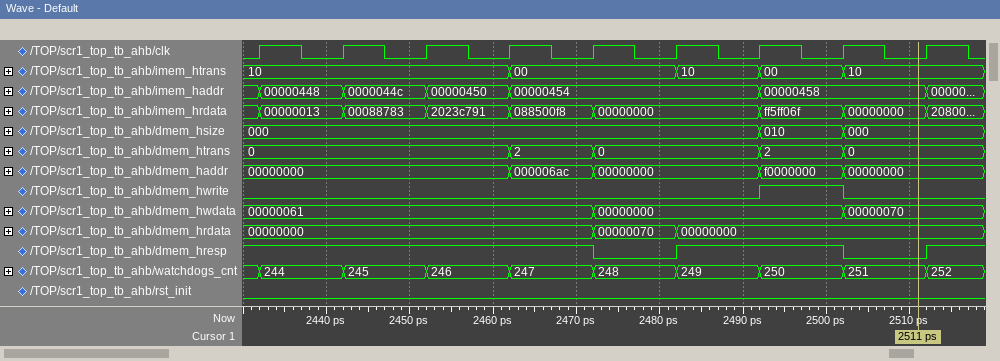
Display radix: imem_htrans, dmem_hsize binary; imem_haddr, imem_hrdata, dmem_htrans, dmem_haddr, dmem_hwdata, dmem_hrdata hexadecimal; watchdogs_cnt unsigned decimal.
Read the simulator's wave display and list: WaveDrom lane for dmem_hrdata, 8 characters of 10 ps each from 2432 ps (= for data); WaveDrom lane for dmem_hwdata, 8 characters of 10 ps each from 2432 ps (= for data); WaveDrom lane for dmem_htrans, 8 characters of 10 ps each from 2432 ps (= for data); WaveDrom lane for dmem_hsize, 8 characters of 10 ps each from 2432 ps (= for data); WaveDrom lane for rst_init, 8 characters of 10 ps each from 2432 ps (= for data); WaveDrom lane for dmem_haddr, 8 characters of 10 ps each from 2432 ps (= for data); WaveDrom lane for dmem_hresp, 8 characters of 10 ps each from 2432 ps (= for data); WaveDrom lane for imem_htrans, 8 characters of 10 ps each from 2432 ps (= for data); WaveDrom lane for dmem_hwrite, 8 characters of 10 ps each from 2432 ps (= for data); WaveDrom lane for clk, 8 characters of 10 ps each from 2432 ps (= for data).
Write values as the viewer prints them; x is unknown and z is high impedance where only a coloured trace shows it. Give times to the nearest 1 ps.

{name: 'dmem_hrdata', wave: '=...==..', data: '00000000 00000070 00000000'}
{name: 'dmem_hwdata', wave: '=...=..=', data: '00000061 00000000 00000070'}
{name: 'dmem_htrans', wave: '=..==.==', data: '0 2 0 2 0'}
{name: 'dmem_hsize', wave: '=.....==', data: '000 010 000'}
{name: 'rst_init', wave: '0.......'}
{name: 'dmem_haddr', wave: '=..==.==', data: '00000000 000006ac 00000000 f0000000 00000000'}
{name: 'dmem_hresp', wave: '1...01.0'}
{name: 'imem_htrans', wave: '=..=.===', data: '10 00 10 00 10'}
{name: 'dmem_hwrite', wave: '0.....10'}
{name: 'clk', wave: 'p.......'}
